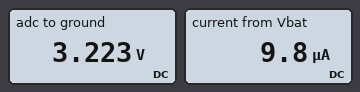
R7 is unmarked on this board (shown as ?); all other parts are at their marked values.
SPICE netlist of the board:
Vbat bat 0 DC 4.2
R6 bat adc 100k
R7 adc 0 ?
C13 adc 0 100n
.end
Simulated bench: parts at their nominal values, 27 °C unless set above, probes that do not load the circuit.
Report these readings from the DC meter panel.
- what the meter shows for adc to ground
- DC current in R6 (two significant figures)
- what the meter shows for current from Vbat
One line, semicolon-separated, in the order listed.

3.223 V; 9.8 µA; 9.8 µA
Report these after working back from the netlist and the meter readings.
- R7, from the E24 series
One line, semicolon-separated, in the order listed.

330 kΩ
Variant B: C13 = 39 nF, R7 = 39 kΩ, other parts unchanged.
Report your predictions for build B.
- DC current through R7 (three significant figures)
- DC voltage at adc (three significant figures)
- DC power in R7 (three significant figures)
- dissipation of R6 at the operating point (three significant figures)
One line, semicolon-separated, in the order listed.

30.2 µA; 1.18 V; 35.6 µW; 91.3 µW
